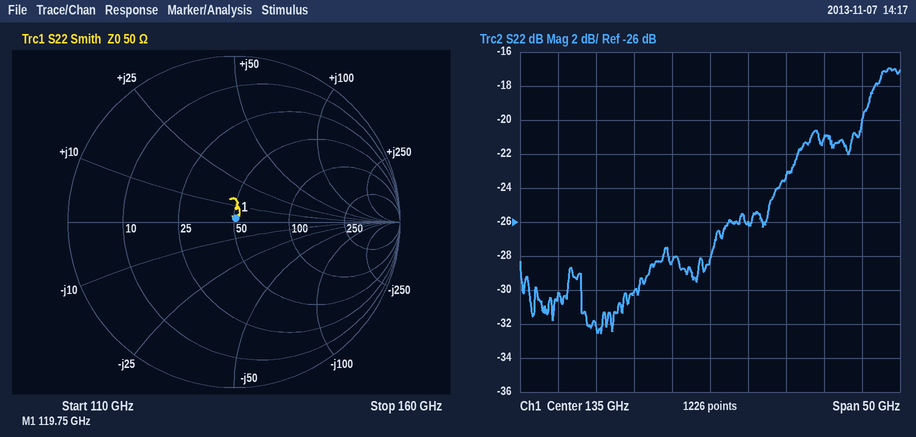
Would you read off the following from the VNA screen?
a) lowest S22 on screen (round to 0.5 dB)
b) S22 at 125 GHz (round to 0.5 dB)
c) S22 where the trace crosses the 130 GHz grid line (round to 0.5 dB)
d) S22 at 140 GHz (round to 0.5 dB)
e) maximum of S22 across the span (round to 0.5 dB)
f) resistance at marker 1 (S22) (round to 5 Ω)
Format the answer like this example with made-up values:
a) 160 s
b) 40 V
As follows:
a) -32.5 dB
b) -30.0 dB
c) -28.5 dB
d) -26.0 dB
e) -17.0 dB
f) 50 Ω
